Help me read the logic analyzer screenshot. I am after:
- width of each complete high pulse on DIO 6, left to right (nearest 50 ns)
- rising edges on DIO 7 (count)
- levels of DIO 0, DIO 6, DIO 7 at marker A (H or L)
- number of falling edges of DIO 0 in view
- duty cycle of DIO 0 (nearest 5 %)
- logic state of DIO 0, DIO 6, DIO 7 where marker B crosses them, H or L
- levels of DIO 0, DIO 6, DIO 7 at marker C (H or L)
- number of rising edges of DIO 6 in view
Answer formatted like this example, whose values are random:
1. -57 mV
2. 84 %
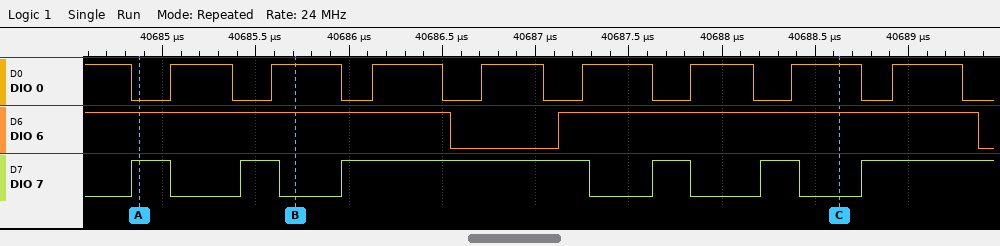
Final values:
1. 2250 ns
2. 6
3. DIO 0=L, DIO 6=H, DIO 7=H
4. 9
5. 65 %
6. DIO 0=H, DIO 6=H, DIO 7=L
7. DIO 0=H, DIO 6=H, DIO 7=L
8. 1
